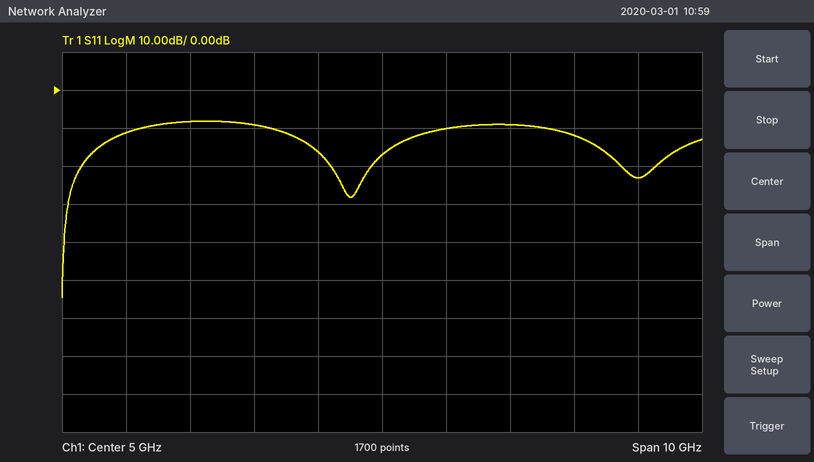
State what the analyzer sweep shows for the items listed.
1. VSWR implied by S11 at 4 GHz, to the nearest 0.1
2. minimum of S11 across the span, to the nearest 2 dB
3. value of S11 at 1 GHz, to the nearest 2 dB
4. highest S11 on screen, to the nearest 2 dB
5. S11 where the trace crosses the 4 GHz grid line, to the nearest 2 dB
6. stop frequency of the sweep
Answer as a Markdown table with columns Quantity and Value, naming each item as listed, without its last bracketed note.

| Quantity | Value |
|---|---|
| VSWR implied by S11 at 4 GHz, to the nearest 0.1 | 1.4 |
| minimum of S11 across the span, to the nearest 2 dB | -54 dB |
| value of S11 at 1 GHz, to the nearest 2 dB | -12 dB |
| highest S11 on screen, to the nearest 2 dB | -8 dB |
| S11 where the trace crosses the 4 GHz grid line, to the nearest 2 dB | -16 dB |
| stop frequency of the sweep | 10 GHz |
